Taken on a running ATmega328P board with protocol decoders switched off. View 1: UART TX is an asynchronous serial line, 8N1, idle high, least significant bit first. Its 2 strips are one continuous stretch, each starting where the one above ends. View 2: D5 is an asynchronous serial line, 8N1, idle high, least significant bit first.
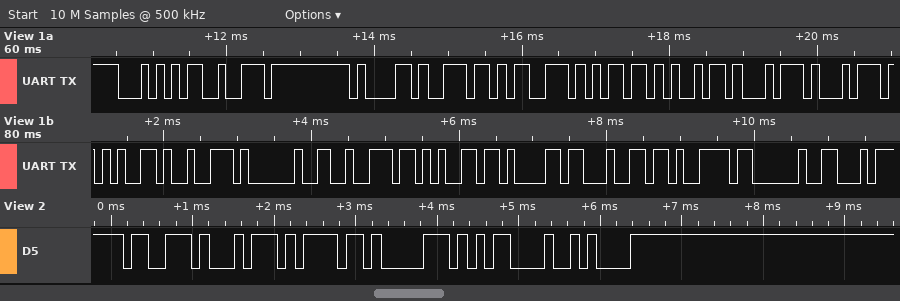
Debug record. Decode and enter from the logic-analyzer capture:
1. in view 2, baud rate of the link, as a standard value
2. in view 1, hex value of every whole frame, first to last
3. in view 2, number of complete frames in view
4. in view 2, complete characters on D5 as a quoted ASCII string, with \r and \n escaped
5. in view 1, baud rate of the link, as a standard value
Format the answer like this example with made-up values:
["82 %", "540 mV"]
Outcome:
["9600 baud", "0x54 0x72 0x61 0x6E 0x73 0x6D 0x69 0x74 0x74 0x65 0x72 0x20 0x72 0x65 0x61 0x64 0x79 0x20", "6", "\"stop\\r\\n\"", "9600 baud"]
